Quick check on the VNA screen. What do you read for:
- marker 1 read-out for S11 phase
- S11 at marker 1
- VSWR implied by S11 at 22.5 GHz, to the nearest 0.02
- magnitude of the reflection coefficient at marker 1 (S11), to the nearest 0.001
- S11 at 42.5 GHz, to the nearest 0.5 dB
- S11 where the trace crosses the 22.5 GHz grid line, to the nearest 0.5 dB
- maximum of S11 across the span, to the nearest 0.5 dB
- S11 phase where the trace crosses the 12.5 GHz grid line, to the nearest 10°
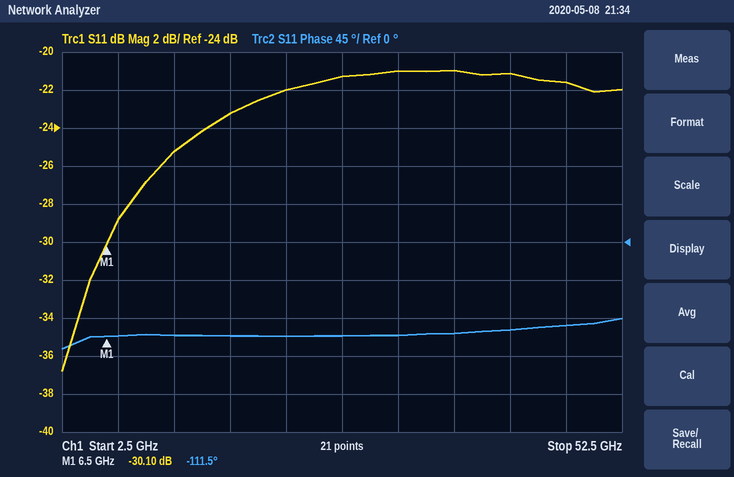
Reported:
-111.5°
-30.10 dB
1.18
0.031
-21.0 dB
-22.0 dB
-21.0 dB
-110°
